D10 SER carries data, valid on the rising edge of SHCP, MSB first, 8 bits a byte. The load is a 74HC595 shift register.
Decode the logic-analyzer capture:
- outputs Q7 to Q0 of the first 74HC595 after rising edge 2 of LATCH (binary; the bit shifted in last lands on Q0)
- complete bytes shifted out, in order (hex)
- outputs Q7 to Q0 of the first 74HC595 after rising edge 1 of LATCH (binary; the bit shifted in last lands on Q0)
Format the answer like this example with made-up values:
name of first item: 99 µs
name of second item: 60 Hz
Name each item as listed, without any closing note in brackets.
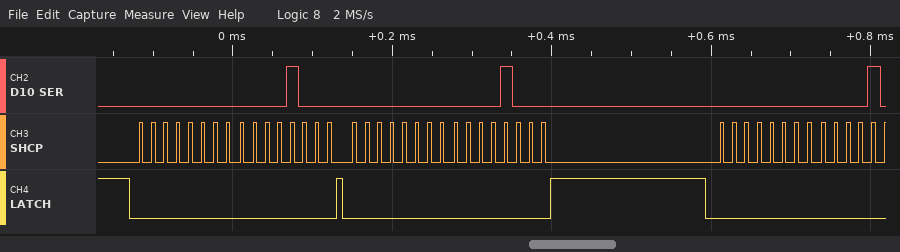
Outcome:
outputs Q7 to Q0 of the first 74HC595 after rising edge 2 of LATCH: 00001000
complete bytes shifted out, in order: 00 08 00 08 00
outputs Q7 to Q0 of the first 74HC595 after rising edge 1 of LATCH: 00001000
